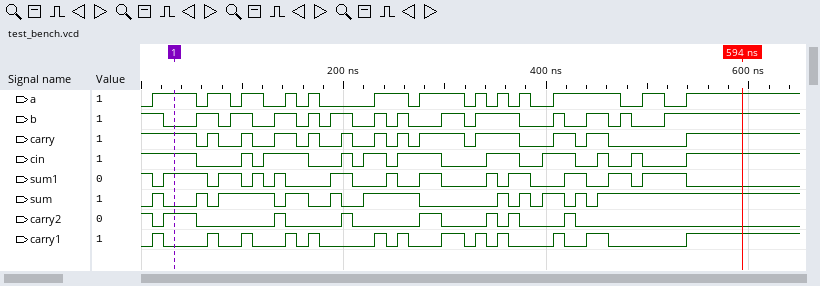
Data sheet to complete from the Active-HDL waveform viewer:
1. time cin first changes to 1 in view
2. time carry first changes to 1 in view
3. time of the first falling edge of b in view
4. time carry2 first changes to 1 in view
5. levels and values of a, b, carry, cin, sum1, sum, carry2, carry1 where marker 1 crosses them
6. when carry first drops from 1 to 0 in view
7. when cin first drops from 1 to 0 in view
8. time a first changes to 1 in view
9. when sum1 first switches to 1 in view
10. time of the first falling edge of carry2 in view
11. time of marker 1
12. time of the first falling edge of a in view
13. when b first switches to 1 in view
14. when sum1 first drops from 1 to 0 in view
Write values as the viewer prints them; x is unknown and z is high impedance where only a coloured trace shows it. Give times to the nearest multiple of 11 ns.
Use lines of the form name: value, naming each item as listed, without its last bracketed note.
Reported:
time cin first changes to 1 in view: 99 ns
time carry first changes to 1 in view: 66 ns
time of the first falling edge of b in view: 22 ns
time carry2 first changes to 1 in view: 22 ns
levels and values of a, b, carry, cin, sum1, sum, carry2, carry1 where marker 1 crosses them: a=1, b=0, carry=1, cin=1, sum1=1, sum=0, carry2=1, carry1=0
when carry first drops from 1 to 0 in view: 55 ns
when cin first drops from 1 to 0 in view: 55 ns
time a first changes to 1 in view: 11 ns
when sum1 first switches to 1 in view: 22 ns
time of the first falling edge of carry2 in view: 11 ns
time of marker 1: 33 ns
time of the first falling edge of a in view: 55 ns
when b first switches to 1 in view: 55 ns
when sum1 first drops from 1 to 0 in view: 11 ns
